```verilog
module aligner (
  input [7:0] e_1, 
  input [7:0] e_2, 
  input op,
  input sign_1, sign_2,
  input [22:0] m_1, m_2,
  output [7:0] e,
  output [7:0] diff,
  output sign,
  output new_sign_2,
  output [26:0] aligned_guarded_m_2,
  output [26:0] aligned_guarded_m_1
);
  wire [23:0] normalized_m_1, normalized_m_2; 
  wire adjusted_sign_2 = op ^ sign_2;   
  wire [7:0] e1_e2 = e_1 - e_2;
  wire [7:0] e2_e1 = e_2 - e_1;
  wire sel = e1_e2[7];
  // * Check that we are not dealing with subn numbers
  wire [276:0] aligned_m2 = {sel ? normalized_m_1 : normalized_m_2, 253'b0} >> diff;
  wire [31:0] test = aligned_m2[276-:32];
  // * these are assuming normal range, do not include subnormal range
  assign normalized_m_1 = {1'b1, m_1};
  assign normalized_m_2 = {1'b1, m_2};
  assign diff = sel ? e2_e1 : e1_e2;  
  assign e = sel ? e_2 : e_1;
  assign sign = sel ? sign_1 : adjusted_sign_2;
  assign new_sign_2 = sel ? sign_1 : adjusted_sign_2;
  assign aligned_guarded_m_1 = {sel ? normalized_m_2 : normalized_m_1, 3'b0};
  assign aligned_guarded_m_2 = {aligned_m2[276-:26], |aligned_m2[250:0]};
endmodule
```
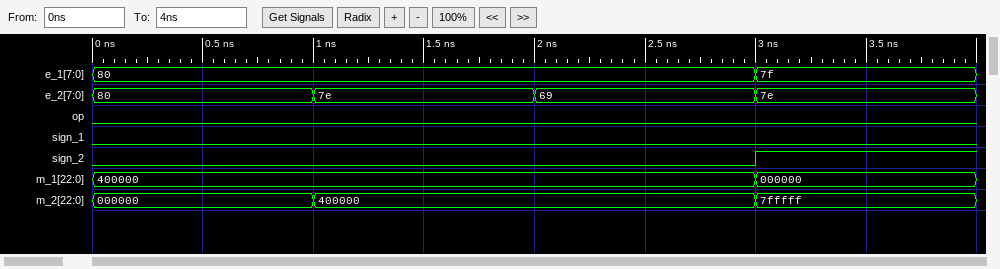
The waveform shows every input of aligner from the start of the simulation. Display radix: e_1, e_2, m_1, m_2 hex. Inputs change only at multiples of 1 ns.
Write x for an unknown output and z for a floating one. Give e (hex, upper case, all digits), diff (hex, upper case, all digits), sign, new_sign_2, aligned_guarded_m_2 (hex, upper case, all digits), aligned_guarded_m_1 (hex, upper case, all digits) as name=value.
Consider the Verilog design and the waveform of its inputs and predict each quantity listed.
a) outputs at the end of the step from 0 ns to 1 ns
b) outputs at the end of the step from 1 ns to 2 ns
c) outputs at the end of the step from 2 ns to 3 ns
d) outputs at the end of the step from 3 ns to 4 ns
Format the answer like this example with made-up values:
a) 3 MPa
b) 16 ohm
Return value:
a) e=80, diff=00, sign=0, new_sign_2=0, aligned_guarded_m_2=4000000, aligned_guarded_m_1=6000000
b) e=80, diff=02, sign=0, new_sign_2=0, aligned_guarded_m_2=1800000, aligned_guarded_m_1=6000000
c) e=80, diff=17, sign=0, new_sign_2=0, aligned_guarded_m_2=000000C, aligned_guarded_m_1=6000000
d) e=7F, diff=01, sign=1, new_sign_2=1, aligned_guarded_m_2=3FFFFFC, aligned_guarded_m_1=4000000
